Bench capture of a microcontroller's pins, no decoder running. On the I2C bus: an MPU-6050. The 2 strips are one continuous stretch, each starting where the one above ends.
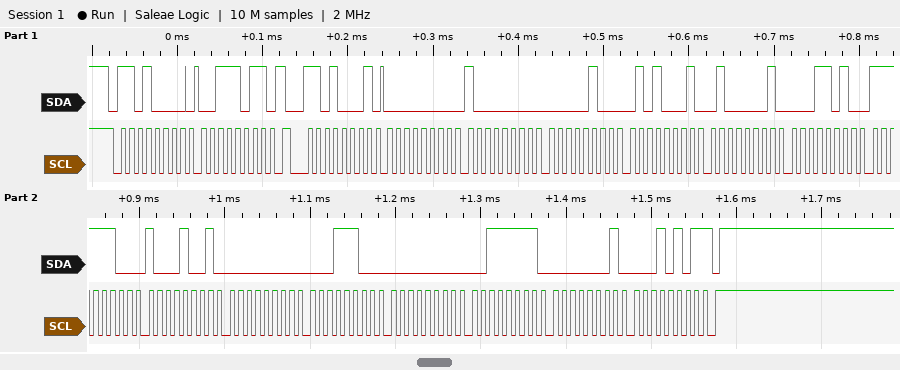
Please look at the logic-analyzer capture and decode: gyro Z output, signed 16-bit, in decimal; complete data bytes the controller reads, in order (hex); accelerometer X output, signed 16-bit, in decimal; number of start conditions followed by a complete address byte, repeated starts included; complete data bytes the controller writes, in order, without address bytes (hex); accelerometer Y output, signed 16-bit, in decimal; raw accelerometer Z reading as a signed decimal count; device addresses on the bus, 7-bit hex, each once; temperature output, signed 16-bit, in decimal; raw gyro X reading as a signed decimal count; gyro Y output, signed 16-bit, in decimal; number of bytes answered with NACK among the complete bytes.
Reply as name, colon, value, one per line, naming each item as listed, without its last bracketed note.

gyro Z output, signed 16-bit, in decimal: 277
complete data bytes the controller reads, in order: 00 80 04 51 41 1A FC 89 00 1C 00 3F 01 15
accelerometer X output, signed 16-bit, in decimal: 128
number of start conditions followed by a complete address byte, repeated starts included: 2
complete data bytes the controller writes, in order, without address bytes: 3B
accelerometer Y output, signed 16-bit, in decimal: 1105
raw accelerometer Z reading as a signed decimal count: 16666
device addresses on the bus, 7-bit hex, each once: 0x68
temperature output, signed 16-bit, in decimal: -887
raw gyro X reading as a signed decimal count: 28
gyro Y output, signed 16-bit, in decimal: 63
number of bytes answered with NACK among the complete bytes: 1
